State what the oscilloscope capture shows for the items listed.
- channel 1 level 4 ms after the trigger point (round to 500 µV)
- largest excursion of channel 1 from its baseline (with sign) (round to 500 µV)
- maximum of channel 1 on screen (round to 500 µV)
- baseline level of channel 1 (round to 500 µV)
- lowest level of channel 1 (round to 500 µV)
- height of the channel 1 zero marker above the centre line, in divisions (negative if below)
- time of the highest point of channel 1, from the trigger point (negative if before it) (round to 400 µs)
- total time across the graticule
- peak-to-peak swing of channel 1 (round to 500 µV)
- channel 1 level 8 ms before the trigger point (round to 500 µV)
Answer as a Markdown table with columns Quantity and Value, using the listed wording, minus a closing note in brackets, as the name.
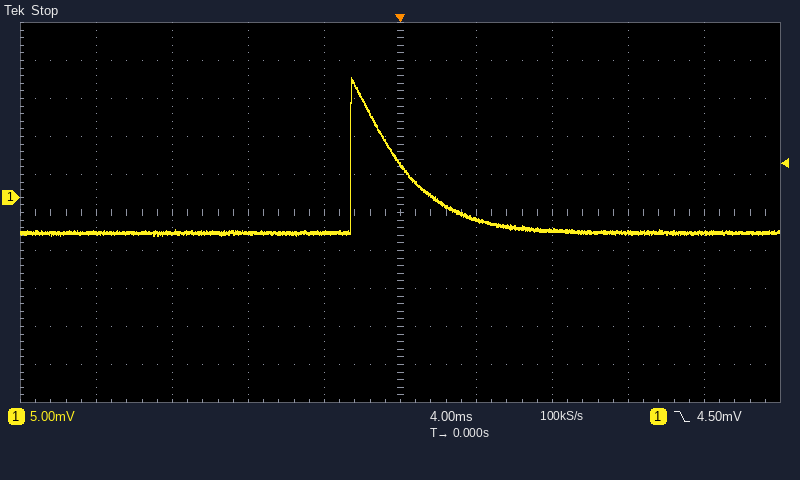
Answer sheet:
| Quantity | Value |
|---|---|
| channel 1 level 4 ms after the trigger point | -3.0 mV |
| largest excursion of channel 1 from its baseline (with sign) | +20.5 mV |
| maximum of channel 1 on screen | 16.0 mV |
| baseline level of channel 1 | -4.5 mV |
| lowest level of channel 1 | -5.0 mV |
| height of the channel 1 zero marker above the centre line, in divisions | +0.4 div |
| time of the highest point of channel 1, from the trigger point (negative if before it) | -2.4 ms |
| total time across the graticule | 40 ms |
| peak-to-peak swing of channel 1 | 21.0 mV |
| channel 1 level 8 ms before the trigger point | -4.5 mV |
